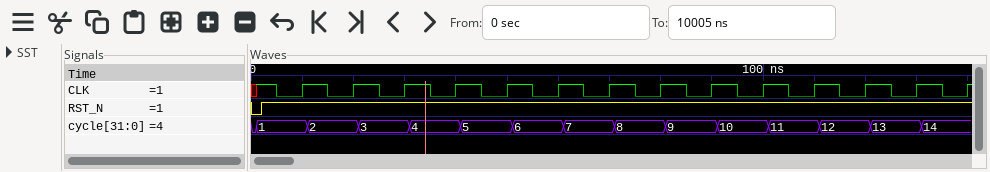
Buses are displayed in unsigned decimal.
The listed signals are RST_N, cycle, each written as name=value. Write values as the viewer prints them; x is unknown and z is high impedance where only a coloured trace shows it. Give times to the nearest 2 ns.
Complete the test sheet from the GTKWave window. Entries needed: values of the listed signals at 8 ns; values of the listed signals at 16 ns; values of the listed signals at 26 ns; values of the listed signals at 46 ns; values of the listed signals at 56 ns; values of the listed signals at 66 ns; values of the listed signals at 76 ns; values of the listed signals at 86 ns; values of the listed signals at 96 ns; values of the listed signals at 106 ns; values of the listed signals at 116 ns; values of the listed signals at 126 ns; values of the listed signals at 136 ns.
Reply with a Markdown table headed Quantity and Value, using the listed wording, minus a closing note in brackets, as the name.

| Quantity | Value |
|---|---|
| values of the listed signals at 8 ns | RST_N=1, cycle=1 |
| values of the listed signals at 16 ns | RST_N=1, cycle=2 |
| values of the listed signals at 26 ns | RST_N=1, cycle=3 |
| values of the listed signals at 46 ns | RST_N=1, cycle=5 |
| values of the listed signals at 56 ns | RST_N=1, cycle=6 |
| values of the listed signals at 66 ns | RST_N=1, cycle=7 |
| values of the listed signals at 76 ns | RST_N=1, cycle=8 |
| values of the listed signals at 86 ns | RST_N=1, cycle=9 |
| values of the listed signals at 96 ns | RST_N=1, cycle=10 |
| values of the listed signals at 106 ns | RST_N=1, cycle=11 |
| values of the listed signals at 116 ns | RST_N=1, cycle=12 |
| values of the listed signals at 126 ns | RST_N=1, cycle=13 |
| values of the listed signals at 136 ns | RST_N=1, cycle=14 |
